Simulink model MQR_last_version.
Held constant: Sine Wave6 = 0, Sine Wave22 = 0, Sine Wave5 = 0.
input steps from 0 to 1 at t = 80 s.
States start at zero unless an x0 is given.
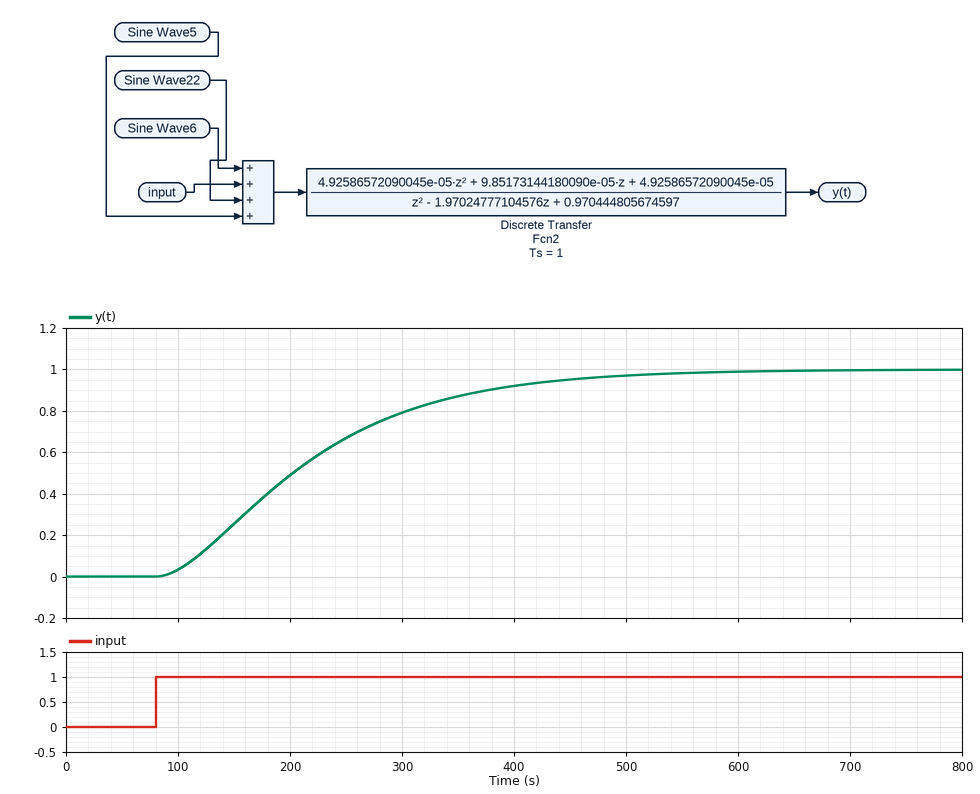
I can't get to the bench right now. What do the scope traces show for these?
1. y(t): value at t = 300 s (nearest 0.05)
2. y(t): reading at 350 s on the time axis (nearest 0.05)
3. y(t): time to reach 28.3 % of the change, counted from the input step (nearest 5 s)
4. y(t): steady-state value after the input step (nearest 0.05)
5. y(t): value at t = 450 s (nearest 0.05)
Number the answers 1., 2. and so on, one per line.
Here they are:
1. 0.80
2. 0.85
3. 75 s
4. 1.00
5. 0.95
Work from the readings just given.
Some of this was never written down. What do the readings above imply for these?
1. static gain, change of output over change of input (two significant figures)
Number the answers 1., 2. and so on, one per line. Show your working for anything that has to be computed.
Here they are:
1. (1 - 0) / (1 - 0) = 1.0
